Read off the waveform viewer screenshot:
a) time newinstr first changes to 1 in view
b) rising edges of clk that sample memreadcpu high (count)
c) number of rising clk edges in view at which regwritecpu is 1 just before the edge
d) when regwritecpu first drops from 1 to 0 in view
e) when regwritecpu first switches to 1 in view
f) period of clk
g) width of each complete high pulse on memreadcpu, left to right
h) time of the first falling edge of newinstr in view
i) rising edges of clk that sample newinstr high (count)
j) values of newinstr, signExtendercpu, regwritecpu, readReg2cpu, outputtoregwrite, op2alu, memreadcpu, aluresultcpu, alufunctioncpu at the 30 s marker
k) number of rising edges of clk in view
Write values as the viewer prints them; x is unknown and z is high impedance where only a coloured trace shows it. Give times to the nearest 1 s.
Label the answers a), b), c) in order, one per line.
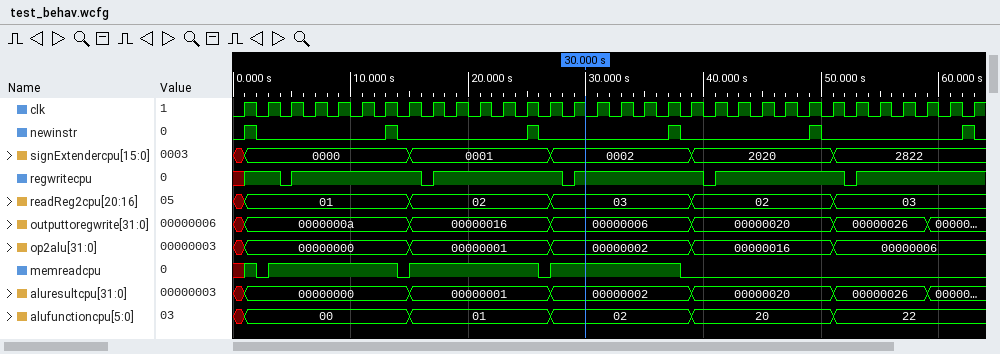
a) 1 s
b) 15
c) 26
d) 4 s
e) 1 s
f) 2 s
g) 11 s, 11 s, 11 s
h) 2 s
i) 1
j) newinstr=0, signExtendercpu=0002, regwritecpu=1, readReg2cpu=03, outputtoregwrite=00000006, op2alu=00000002, memreadcpu=1, aluresultcpu=00000002, alufunctioncpu=02
k) 32
